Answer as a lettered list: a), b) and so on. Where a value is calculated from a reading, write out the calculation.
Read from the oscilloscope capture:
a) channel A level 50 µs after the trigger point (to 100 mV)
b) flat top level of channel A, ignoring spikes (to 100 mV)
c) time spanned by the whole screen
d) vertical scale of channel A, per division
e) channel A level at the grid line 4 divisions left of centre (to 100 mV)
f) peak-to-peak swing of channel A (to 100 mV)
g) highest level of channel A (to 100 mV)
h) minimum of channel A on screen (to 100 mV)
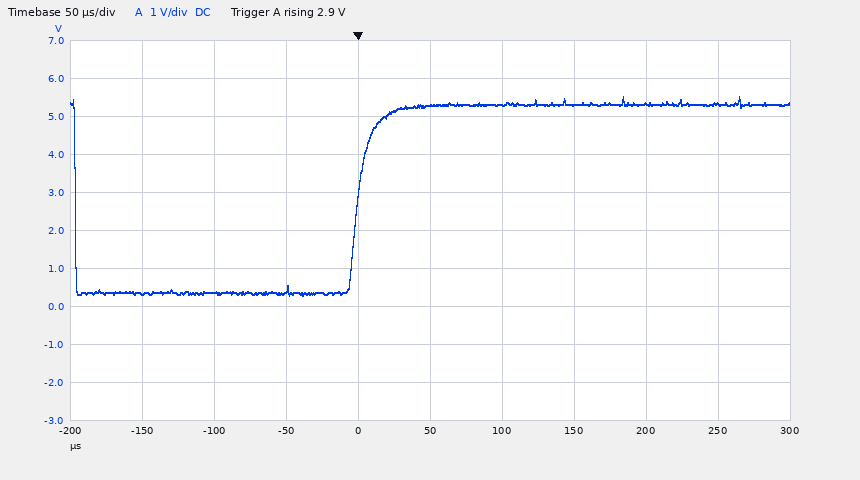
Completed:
a) 5.3 V
b) 5.3 V
c) 500 µs
d) 1 V
e) 300 mV
f) 5.5 V − (300 mV) = 5.2 V
g) 5.5 V
h) 300 mV
